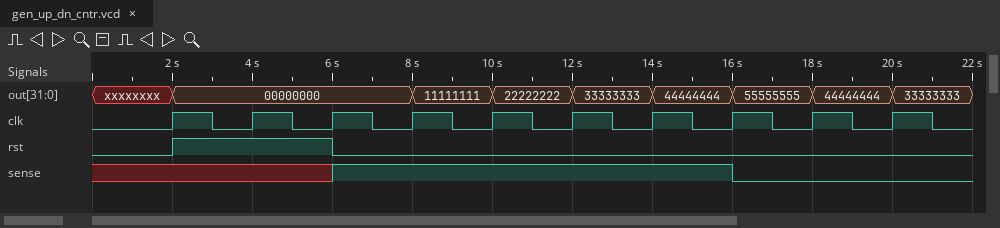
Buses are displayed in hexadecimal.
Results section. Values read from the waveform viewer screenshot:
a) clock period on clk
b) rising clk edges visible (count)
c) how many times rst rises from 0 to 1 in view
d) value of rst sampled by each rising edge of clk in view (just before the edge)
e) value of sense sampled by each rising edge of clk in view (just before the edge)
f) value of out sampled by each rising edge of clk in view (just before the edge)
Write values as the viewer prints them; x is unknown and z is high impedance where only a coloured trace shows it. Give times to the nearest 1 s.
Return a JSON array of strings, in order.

["2 s", "10", "1", "0 1 1 0 0 0 0 0 0 0", "x x x 1 1 1 1 1 0 0", "xxxxxxxx, 00000000, 00000000, 00000000, 11111111, 22222222, 33333333, 44444444, 55555555, 44444444"]
